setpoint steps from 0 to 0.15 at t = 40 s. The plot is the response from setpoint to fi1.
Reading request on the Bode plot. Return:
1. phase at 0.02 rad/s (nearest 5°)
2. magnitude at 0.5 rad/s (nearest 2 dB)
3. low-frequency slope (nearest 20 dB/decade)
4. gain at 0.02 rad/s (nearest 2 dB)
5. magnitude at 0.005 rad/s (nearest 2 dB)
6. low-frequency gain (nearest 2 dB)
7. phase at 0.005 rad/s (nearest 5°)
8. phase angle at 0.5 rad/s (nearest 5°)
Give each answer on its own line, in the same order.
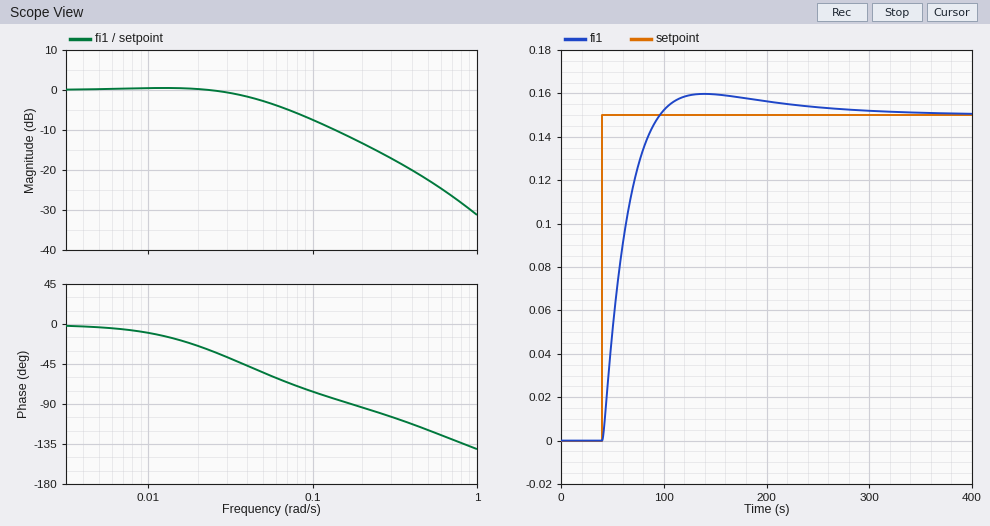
-25°
-22 dB
0 dB/decade
0 dB
0 dB
0 dB
-5°
-120°
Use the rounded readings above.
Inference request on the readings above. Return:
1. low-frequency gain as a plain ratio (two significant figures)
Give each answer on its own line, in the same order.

1.0
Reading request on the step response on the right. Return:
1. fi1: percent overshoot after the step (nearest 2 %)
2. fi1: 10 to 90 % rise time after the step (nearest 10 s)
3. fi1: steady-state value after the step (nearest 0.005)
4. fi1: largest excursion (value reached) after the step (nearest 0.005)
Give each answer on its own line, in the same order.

6 %
40 s
0.150
0.160
